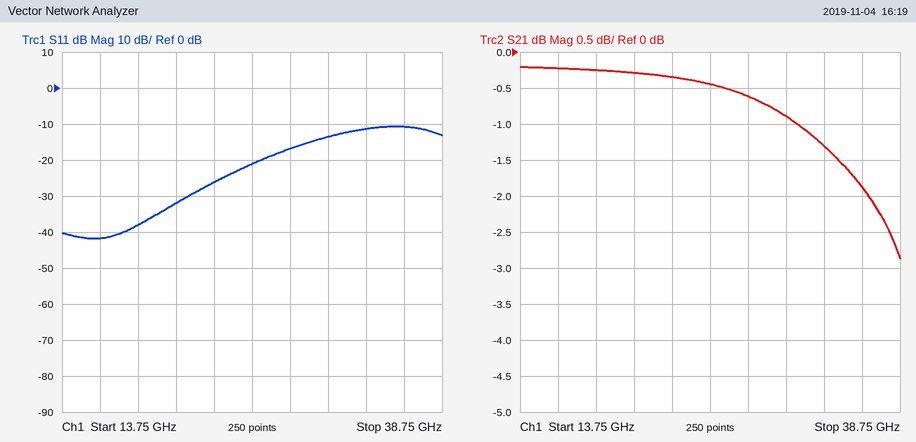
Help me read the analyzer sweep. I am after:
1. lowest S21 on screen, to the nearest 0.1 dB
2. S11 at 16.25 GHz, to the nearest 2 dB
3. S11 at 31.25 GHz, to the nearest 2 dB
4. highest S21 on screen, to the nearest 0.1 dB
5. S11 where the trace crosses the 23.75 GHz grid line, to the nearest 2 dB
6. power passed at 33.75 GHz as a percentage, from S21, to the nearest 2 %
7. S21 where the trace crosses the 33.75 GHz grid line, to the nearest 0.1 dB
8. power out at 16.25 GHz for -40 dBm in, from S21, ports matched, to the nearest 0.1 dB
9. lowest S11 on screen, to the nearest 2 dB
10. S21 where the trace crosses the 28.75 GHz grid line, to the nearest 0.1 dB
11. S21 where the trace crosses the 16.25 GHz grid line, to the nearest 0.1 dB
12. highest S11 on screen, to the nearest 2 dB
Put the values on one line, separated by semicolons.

-2.9 dB; -42 dB; -14 dB; -0.2 dB; -26 dB; 74 %; -1.3 dB; -40.2 dBm; -42 dB; -0.6 dB; -0.2 dB; -10 dB
